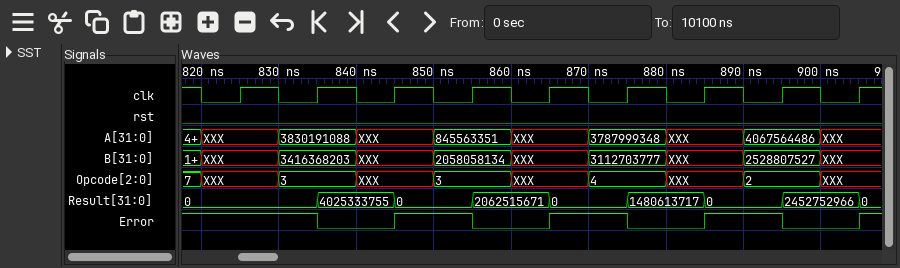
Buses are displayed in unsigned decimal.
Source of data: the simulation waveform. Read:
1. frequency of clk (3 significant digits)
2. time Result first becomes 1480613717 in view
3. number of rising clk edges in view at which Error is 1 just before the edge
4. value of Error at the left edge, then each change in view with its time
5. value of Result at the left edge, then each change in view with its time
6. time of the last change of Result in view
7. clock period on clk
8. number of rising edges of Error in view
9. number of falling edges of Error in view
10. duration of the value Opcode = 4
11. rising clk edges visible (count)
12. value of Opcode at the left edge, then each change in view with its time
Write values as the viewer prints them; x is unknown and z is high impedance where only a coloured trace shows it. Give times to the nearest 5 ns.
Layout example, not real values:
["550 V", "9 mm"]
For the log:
["100 MHz", "875 ns", "5", "1, 0 at 835 ns, 1 at 845 ns, 0 at 855 ns, 1 at 865 ns, 0 at 875 ns, 1 at 885 ns, 0 at 895 ns, 1 at 905 ns", "0, 4025333755 at 835 ns, 0 at 845 ns, 2062515671 at 855 ns, 0 at 865 ns, 1480613717 at 875 ns, 0 at 885 ns, 2452752966 at 895 ns, 0 at 905 ns", "905 ns", "10 ns", "4", "4", "10 ns", "9", "7, XXX at 820 ns, 3 at 830 ns, XXX at 840 ns, 3 at 850 ns, XXX at 860 ns, 4 at 870 ns, XXX at 880 ns, 2 at 890 ns, XXX at 900 ns"]
